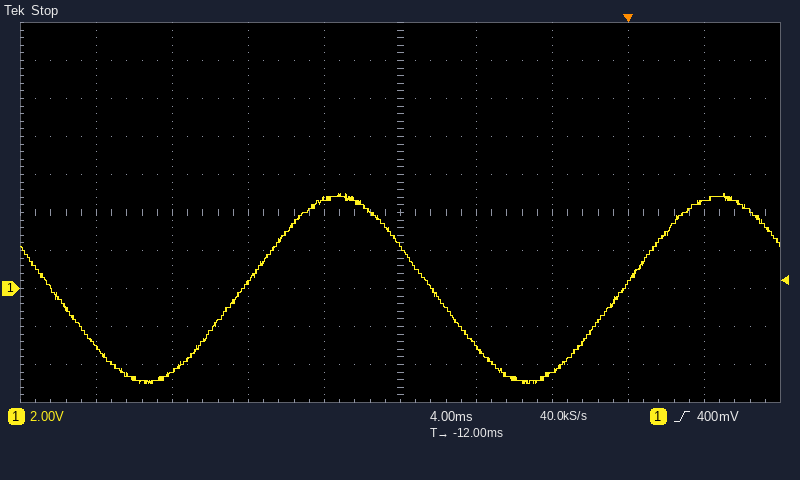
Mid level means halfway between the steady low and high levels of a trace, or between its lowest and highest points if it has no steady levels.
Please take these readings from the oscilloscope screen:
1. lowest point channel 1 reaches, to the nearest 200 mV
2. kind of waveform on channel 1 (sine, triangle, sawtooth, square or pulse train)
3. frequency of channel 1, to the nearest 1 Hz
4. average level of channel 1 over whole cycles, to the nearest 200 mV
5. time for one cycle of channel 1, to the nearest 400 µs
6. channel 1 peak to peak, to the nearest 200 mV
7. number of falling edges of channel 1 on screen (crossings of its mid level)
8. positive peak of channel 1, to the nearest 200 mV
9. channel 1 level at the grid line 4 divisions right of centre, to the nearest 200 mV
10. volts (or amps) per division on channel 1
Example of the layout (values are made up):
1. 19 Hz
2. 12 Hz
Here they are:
1. -5.0 V
2. sine
3. 50 Hz
4. 0.0 V
5. 20.0 ms
6. 10.0 V
7. 2
8. 5.0 V
9. 4.6 V
10. 2 V
